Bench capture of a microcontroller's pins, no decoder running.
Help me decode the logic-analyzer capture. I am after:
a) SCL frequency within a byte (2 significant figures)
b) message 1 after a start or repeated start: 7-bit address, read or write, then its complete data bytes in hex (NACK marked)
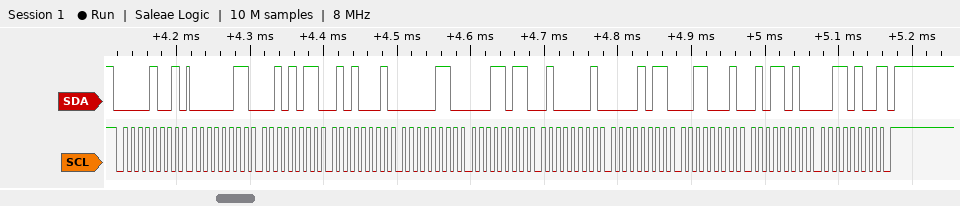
100 kHz
0x04 read: 03 2B 51 06 1B 41 0B 31 5A 34 NACK
